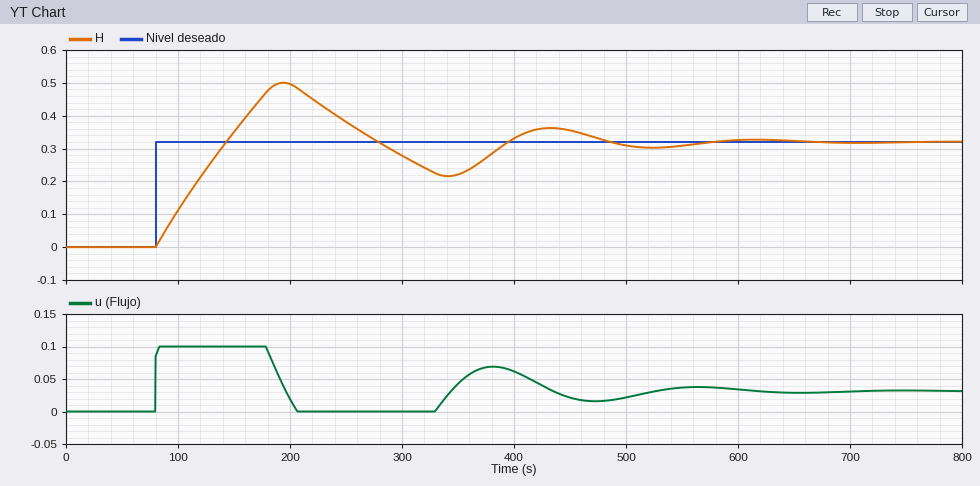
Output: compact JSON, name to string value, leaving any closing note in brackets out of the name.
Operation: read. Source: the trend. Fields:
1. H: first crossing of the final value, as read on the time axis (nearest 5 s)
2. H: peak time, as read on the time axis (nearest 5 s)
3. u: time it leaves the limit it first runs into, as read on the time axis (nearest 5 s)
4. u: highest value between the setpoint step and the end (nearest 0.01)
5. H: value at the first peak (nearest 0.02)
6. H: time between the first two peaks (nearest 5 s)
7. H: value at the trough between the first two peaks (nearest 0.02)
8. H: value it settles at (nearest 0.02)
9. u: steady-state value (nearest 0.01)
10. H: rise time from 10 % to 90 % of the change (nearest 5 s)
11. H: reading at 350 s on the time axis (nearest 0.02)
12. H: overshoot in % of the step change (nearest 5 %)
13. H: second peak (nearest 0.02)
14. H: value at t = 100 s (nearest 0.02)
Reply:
{"H: first crossing of the final value, as read on the time axis": "145 s", "H: peak time, as read on the time axis": "195 s", "u: time it leaves the limit it first runs into, as read on the time axis": "180 s", "u: highest value between the setpoint step and the end": "0.10", "H: value at the first peak": "0.50", "H: time between the first two peaks": "240 s", "H: value at the trough between the first two peaks": "0.22", "H: value it settles at": "0.32", "u: steady-state value": "0.03", "H: rise time from 10 % to 90 % of the change": "50 s", "H: reading at 350 s on the time axis": "0.22", "H: overshoot in % of the step change": "55 %", "H: second peak": "0.36", "H: value at t = 100 s": "0.12"}
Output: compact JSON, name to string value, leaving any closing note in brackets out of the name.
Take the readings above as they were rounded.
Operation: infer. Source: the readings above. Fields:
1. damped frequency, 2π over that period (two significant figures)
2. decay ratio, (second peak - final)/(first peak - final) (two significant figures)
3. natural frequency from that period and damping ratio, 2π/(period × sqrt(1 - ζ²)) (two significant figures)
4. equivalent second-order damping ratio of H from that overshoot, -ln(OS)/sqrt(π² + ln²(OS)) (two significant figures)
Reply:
{"damped frequency, 2π over that period": "0.026 rad/s", "decay ratio, (second peak - final)/(first peak - final)": "0.22", "natural frequency from that period and damping ratio, 2π/(period × sqrt(1 - ζ²))": "0.027 rad/s", "equivalent second-order damping ratio of H from that overshoot, -ln(OS)/sqrt(π² + ln²(OS))": "0.19"}
